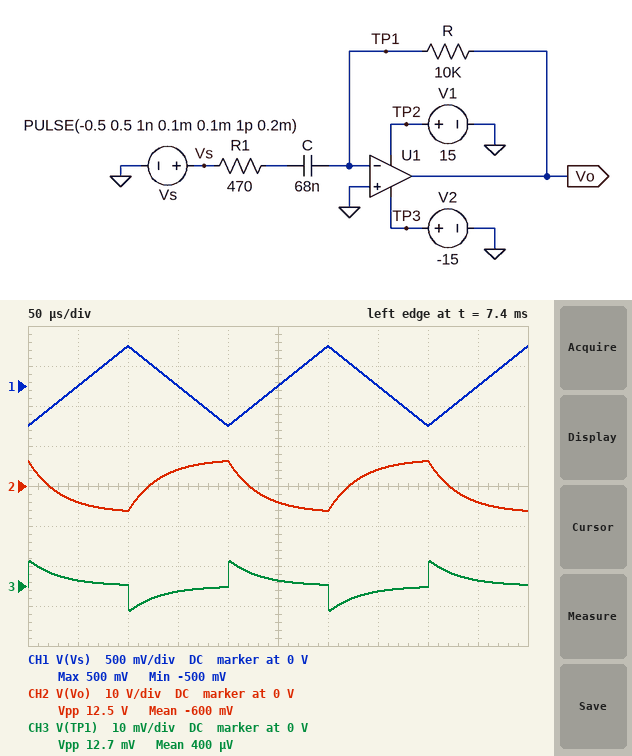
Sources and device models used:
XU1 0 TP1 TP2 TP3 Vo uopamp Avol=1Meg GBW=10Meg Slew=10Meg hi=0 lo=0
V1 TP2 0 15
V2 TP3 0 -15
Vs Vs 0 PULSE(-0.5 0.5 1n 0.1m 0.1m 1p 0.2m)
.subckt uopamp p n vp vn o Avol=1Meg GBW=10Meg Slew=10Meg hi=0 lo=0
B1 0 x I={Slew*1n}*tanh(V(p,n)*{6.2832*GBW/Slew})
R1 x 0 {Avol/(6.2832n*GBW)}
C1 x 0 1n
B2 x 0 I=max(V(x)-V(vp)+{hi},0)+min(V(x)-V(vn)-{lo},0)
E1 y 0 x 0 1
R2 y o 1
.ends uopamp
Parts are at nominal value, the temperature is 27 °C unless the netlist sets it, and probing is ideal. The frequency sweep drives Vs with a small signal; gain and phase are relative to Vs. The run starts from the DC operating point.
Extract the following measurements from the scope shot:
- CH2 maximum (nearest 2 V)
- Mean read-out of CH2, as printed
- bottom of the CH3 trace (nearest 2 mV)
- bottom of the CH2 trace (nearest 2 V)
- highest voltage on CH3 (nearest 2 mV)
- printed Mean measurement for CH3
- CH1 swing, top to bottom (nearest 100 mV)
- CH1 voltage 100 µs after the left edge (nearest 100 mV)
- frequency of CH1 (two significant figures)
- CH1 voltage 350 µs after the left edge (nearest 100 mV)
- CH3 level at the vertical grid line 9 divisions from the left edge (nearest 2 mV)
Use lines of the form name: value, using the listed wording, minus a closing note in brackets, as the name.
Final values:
CH2 maximum: 6 V
Mean read-out of CH2, as printed: -600 mV
bottom of the CH3 trace: -6 mV
bottom of the CH2 trace: -6 V
highest voltage on CH3: 6 mV
printed Mean measurement for CH3: 400 µV
CH1 swing, top to bottom: 1.0 V
CH1 voltage 100 µs after the left edge: 500 mV
frequency of CH1: 5.0 kHz
CH1 voltage 350 µs after the left edge: 0 V
CH3 level at the vertical grid line 9 divisions from the left edge: 2 mV
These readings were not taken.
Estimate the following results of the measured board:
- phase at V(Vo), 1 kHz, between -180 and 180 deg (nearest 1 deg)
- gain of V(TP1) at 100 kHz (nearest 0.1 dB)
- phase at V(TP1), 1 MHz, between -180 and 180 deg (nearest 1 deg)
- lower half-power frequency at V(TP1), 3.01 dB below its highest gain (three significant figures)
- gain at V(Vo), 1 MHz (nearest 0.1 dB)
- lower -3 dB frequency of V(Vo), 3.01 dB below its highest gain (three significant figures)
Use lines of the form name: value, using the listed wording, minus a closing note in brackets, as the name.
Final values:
phase at V(Vo), 1 kHz, between -180 and 180 deg: -101 deg
gain of V(TP1) at 100 kHz: -13.6 dB
phase at V(TP1), 1 MHz, between -180 and 180 deg: 24 deg
lower half-power frequency at V(TP1), 3.01 dB below its highest gain: 444 kHz
gain at V(Vo), 1 MHz: 18.8 dB
lower -3 dB frequency of V(Vo), 3.01 dB below its highest gain: 4.92 kHz
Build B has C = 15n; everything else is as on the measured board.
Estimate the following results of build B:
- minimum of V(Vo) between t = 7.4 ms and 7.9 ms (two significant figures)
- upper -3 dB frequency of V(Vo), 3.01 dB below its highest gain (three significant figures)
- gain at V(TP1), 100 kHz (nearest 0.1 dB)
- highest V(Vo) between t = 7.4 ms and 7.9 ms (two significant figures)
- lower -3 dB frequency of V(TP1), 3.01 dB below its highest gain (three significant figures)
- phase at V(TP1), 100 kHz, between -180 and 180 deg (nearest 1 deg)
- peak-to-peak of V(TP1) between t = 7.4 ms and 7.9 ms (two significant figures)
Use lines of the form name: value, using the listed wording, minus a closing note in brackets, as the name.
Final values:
minimum of V(Vo) between t = 7.4 ms and 7.9 ms: -1.5 V
upper -3 dB frequency of V(Vo), 3.01 dB below its highest gain: 471 kHz
gain at V(TP1), 100 kHz: -13.5 dB
highest V(Vo) between t = 7.4 ms and 7.9 ms: 1.5 V
lower -3 dB frequency of V(TP1), 3.01 dB below its highest gain: 427 kHz
phase at V(TP1), 100 kHz, between -180 and 180 deg: 90 deg
peak-to-peak of V(TP1) between t = 7.4 ms and 7.9 ms: 12 mV
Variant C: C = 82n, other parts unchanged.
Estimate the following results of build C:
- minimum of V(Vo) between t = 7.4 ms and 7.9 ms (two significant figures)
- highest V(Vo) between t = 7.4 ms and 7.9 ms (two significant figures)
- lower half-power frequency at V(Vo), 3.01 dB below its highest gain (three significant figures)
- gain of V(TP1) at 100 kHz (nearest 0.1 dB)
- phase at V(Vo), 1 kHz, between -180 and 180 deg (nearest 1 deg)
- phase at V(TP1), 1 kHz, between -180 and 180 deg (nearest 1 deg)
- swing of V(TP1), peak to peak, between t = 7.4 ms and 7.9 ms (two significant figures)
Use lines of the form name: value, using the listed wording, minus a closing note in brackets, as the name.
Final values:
minimum of V(Vo) between t = 7.4 ms and 7.9 ms: -7.1 V
highest V(Vo) between t = 7.4 ms and 7.9 ms: 7.1 V
lower half-power frequency at V(Vo), 3.01 dB below its highest gain: 4.09 kHz
gain of V(TP1) at 100 kHz: -13.6 dB
phase at V(Vo), 1 kHz, between -180 and 180 deg: -104 deg
phase at V(TP1), 1 kHz, between -180 and 180 deg: 166 deg
swing of V(TP1), peak to peak, between t = 7.4 ms and 7.9 ms: 12 mV
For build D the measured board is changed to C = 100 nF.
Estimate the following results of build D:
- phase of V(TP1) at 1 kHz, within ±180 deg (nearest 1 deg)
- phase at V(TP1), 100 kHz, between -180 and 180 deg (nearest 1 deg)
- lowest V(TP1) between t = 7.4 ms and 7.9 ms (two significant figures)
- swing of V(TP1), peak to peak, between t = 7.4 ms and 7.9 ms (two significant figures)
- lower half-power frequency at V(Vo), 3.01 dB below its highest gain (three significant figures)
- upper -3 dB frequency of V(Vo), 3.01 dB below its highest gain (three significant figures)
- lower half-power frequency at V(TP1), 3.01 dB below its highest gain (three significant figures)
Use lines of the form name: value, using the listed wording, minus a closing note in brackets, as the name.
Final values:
phase of V(TP1) at 1 kHz, within ±180 deg: 163 deg
phase at V(TP1), 100 kHz, between -180 and 180 deg: 79 deg
lowest V(TP1) between t = 7.4 ms and 7.9 ms: -5.9 mV
swing of V(TP1), peak to peak, between t = 7.4 ms and 7.9 ms: 12 mV
lower half-power frequency at V(Vo), 3.01 dB below its highest gain: 3.36 kHz
upper -3 dB frequency of V(Vo), 3.01 dB below its highest gain: 452 kHz
lower half-power frequency at V(TP1), 3.01 dB below its highest gain: 446 kHz
